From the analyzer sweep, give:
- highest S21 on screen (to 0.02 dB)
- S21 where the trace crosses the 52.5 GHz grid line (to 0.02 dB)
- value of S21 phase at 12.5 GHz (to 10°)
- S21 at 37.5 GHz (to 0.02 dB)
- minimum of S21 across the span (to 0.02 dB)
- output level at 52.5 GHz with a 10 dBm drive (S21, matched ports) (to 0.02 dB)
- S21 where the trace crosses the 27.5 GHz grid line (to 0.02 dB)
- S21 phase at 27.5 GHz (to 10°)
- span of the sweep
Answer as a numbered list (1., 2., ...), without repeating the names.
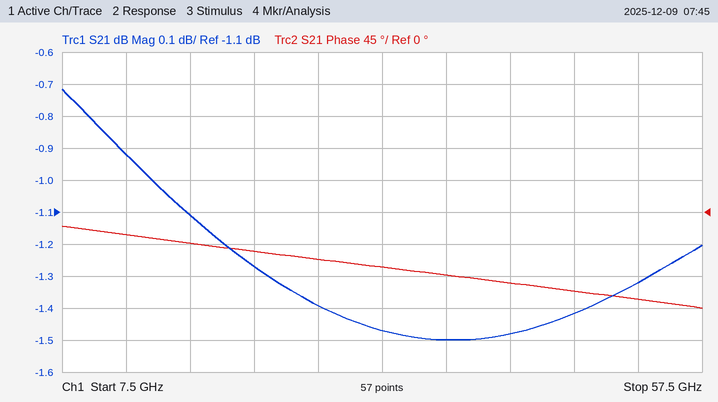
1. -0.72 dB
2. -1.32 dB
3. -30°
4. -1.50 dB
5. -1.50 dB
6. 8.68 dBm
7. -1.40 dB
8. -70°
9. 50 GHz
